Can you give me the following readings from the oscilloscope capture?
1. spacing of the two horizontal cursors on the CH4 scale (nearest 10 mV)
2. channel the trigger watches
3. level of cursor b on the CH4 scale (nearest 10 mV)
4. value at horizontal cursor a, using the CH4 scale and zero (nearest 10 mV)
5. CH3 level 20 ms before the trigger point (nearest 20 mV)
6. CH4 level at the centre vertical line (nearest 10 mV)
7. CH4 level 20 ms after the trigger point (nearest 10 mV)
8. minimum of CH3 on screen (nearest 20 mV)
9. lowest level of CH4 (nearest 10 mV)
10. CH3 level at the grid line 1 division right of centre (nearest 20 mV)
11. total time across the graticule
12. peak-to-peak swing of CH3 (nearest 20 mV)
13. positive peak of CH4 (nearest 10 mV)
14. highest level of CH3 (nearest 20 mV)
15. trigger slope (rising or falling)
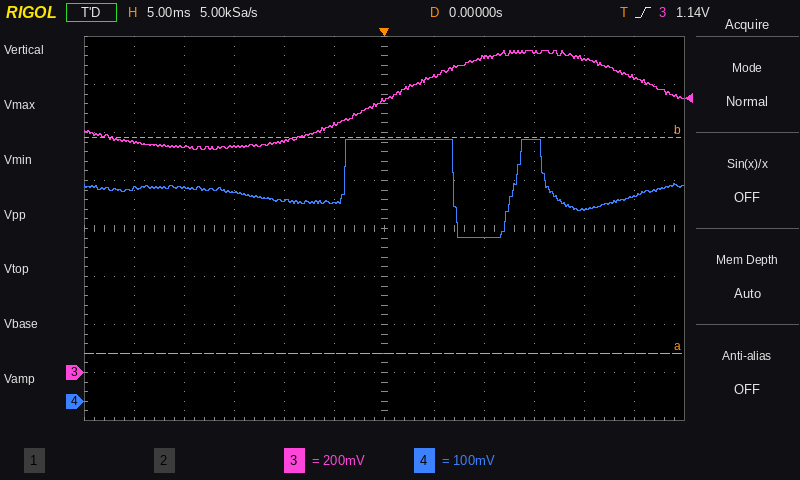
450 mV
CH3
550 mV
100 mV
940 mV
550 mV
400 mV
920 mV
340 mV
1.24 V
60 ms
420 mV
550 mV
1.34 V
rising
